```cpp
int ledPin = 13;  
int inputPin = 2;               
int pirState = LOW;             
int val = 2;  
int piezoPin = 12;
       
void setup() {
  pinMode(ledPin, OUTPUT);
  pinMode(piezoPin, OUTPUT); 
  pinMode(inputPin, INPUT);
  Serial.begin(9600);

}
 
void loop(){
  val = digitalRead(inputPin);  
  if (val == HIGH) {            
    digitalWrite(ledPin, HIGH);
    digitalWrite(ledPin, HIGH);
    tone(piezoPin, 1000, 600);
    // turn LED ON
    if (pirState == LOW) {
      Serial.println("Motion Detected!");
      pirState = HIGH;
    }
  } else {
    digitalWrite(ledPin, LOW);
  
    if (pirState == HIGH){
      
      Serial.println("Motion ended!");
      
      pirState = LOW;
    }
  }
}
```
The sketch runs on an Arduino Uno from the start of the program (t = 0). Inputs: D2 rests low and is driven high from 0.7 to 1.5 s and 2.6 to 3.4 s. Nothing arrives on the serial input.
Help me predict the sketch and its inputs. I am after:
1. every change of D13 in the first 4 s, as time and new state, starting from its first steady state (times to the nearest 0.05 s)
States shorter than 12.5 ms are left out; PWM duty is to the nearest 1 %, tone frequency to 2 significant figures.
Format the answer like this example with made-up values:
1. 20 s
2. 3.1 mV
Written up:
1. 0 s low; 0.7 s high; 1.5 s low; 2.6 s high; 3.4 s low
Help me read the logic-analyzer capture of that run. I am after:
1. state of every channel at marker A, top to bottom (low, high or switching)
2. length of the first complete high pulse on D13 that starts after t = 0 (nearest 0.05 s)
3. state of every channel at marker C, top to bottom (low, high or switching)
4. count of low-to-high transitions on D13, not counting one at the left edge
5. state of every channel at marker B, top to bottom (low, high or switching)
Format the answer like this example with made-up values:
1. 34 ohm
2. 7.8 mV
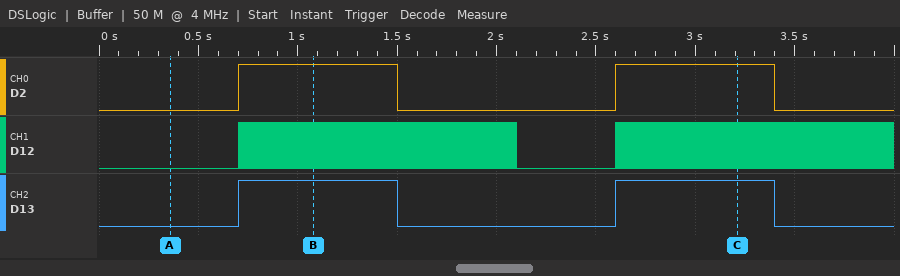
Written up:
1. D2 low, D12 low, D13 low
2. 0.80 s
3. D2 high, D12 switching, D13 high
4. 2
5. D2 high, D12 switching, D13 high
